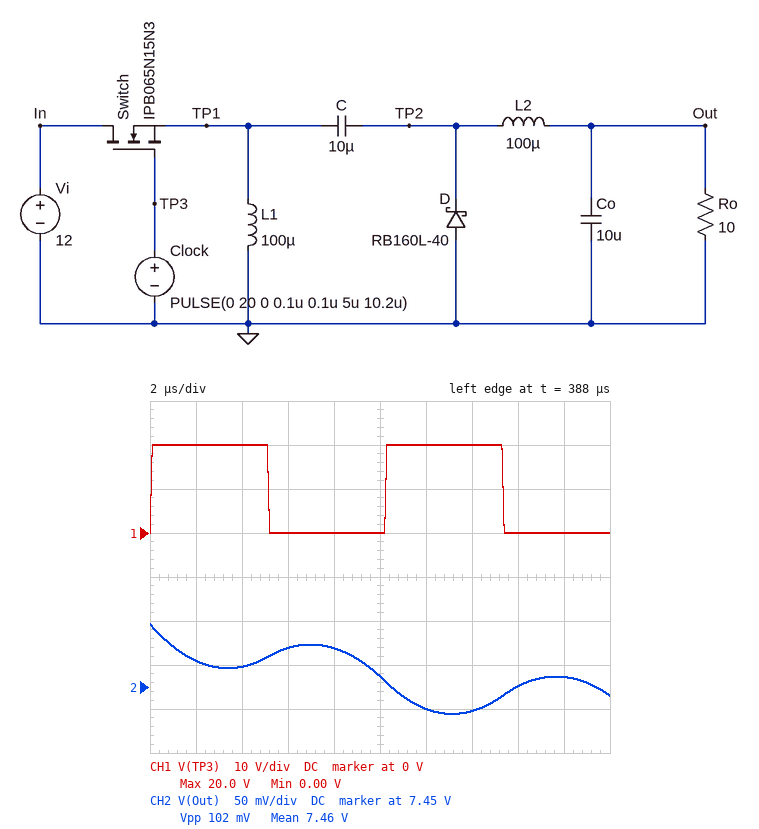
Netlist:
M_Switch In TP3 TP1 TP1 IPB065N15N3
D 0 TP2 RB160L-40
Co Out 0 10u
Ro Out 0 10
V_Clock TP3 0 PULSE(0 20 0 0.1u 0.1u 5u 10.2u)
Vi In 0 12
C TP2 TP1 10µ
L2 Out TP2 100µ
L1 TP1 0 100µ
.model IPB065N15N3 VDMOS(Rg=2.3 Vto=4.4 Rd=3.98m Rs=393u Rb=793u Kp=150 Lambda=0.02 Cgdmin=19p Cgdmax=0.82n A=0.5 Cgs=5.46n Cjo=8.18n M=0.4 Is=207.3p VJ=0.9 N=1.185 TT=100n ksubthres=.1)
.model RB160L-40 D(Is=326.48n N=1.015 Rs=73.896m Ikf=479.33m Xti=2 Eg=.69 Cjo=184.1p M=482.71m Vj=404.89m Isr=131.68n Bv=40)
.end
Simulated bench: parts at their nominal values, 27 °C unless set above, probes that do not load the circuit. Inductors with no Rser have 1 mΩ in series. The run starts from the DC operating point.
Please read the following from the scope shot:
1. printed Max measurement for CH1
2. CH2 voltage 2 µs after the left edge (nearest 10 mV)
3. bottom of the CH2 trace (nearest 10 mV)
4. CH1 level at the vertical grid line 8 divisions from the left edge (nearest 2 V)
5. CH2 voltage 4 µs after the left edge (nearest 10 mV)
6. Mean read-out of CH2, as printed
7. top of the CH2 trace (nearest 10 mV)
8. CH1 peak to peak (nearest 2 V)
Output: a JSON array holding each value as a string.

["20.0 V", "7.48 V", "7.42 V", "0 V", "7.47 V", "7.46 V", "7.52 V", "20 V"]
